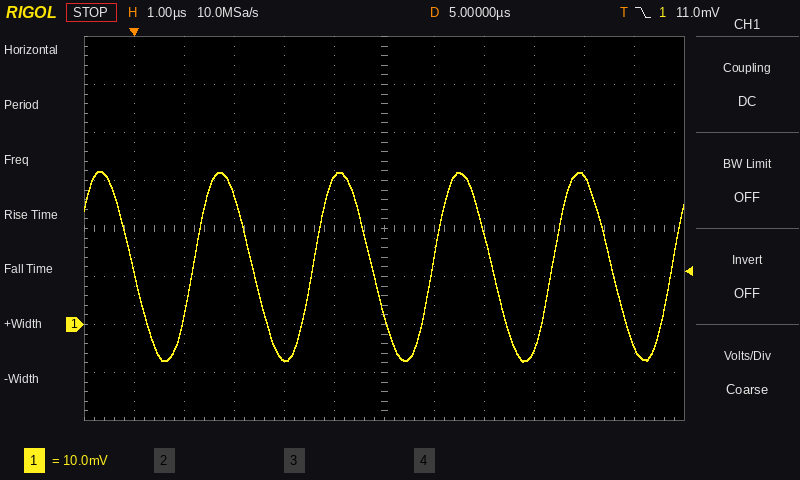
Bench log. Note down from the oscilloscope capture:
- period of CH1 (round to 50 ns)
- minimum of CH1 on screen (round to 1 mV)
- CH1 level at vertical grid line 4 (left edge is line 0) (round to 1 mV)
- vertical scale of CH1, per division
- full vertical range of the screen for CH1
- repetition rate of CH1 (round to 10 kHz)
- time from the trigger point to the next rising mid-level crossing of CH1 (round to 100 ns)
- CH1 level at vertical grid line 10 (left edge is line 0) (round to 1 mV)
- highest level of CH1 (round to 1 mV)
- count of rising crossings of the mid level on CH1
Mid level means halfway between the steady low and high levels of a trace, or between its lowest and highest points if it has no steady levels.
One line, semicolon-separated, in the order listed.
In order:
2.40 µs; -8 mV; -7 mV; 10 mV; 80 mV; 420 kHz; 1.2 µs; 31 mV; 32 mV; 5
